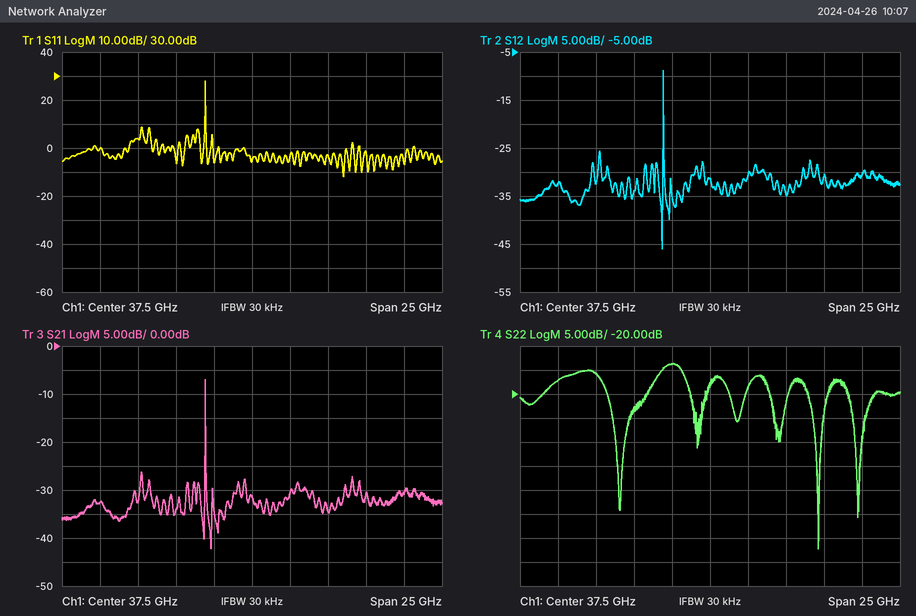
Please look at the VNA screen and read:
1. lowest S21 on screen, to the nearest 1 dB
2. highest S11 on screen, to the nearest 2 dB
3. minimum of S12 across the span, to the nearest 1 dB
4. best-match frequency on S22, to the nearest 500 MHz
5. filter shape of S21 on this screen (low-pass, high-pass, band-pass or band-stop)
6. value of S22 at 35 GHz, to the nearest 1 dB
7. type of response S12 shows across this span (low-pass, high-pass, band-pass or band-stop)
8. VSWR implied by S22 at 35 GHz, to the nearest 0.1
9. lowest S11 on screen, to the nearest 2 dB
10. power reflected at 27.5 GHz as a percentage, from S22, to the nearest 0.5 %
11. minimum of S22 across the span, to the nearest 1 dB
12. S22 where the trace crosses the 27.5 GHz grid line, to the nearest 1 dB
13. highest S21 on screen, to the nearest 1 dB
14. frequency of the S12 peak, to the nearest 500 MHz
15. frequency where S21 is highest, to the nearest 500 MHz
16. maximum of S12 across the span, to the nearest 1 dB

-42 dB
28 dB
-46 dB
44.5 GHz
band-pass
-14 dB
band-pass
1.5
-12 dB
2.0 %
-52 dB
-17 dB
-7 dB
34.5 GHz
34.5 GHz
-9 dB
